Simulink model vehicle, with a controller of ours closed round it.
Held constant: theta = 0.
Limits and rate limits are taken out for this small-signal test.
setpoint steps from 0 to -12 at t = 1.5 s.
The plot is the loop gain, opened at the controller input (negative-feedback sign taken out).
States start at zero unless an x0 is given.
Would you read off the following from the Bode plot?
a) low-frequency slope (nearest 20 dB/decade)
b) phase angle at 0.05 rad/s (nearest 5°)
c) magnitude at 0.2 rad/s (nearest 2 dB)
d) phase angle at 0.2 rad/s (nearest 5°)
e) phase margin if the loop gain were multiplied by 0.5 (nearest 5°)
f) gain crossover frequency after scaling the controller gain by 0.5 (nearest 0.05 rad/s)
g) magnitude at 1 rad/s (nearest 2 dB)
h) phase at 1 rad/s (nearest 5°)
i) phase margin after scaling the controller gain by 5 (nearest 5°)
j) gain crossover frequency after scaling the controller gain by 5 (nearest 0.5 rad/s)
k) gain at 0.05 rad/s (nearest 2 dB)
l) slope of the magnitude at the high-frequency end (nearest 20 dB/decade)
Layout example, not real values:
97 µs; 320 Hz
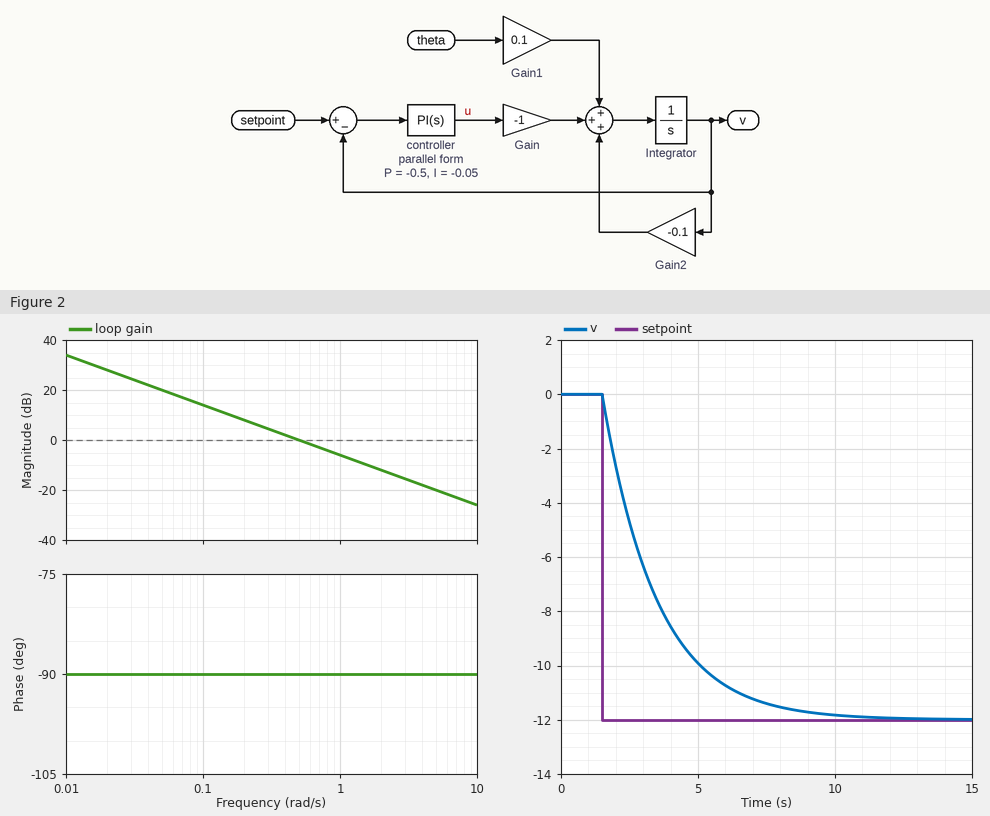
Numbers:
-20 dB/decade; -90°; 8 dB; -90°; 90°; 0.25 rad/s; -6 dB; -90°; 90°; 2.5 rad/s; 20 dB; -20 dB/decade
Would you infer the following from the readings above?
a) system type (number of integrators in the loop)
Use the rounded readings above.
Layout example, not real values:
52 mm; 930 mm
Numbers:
1
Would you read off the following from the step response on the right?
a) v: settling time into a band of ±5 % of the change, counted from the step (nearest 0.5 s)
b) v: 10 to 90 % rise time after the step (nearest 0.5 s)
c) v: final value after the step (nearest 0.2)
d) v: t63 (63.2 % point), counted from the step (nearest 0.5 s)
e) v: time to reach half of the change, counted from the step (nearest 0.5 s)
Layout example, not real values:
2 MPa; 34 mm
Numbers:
6.0 s; 4.5 s; -12.0; 2.0 s; 1.5 s
